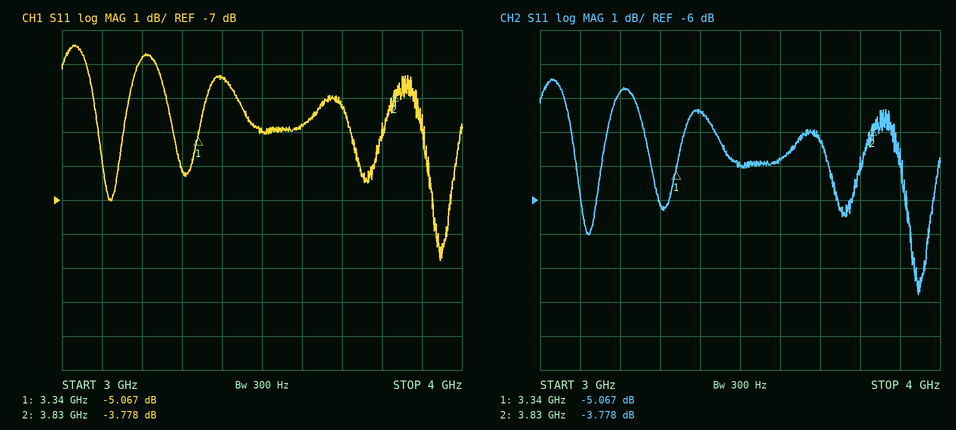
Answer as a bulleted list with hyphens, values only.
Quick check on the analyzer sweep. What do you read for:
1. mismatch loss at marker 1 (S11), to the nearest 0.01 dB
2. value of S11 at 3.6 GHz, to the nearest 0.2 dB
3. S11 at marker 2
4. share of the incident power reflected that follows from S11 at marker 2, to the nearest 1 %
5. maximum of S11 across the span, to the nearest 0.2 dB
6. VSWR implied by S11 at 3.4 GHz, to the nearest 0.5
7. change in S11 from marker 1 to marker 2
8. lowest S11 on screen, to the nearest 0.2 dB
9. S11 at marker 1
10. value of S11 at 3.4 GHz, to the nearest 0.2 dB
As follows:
- 1.62 dB
- -4.8 dB
- -3.778 dB
- 42 %
- -2.4 dB
- 5.0
- 1.289 dB
- -8.8 dB
- -5.067 dB
- -3.4 dB
